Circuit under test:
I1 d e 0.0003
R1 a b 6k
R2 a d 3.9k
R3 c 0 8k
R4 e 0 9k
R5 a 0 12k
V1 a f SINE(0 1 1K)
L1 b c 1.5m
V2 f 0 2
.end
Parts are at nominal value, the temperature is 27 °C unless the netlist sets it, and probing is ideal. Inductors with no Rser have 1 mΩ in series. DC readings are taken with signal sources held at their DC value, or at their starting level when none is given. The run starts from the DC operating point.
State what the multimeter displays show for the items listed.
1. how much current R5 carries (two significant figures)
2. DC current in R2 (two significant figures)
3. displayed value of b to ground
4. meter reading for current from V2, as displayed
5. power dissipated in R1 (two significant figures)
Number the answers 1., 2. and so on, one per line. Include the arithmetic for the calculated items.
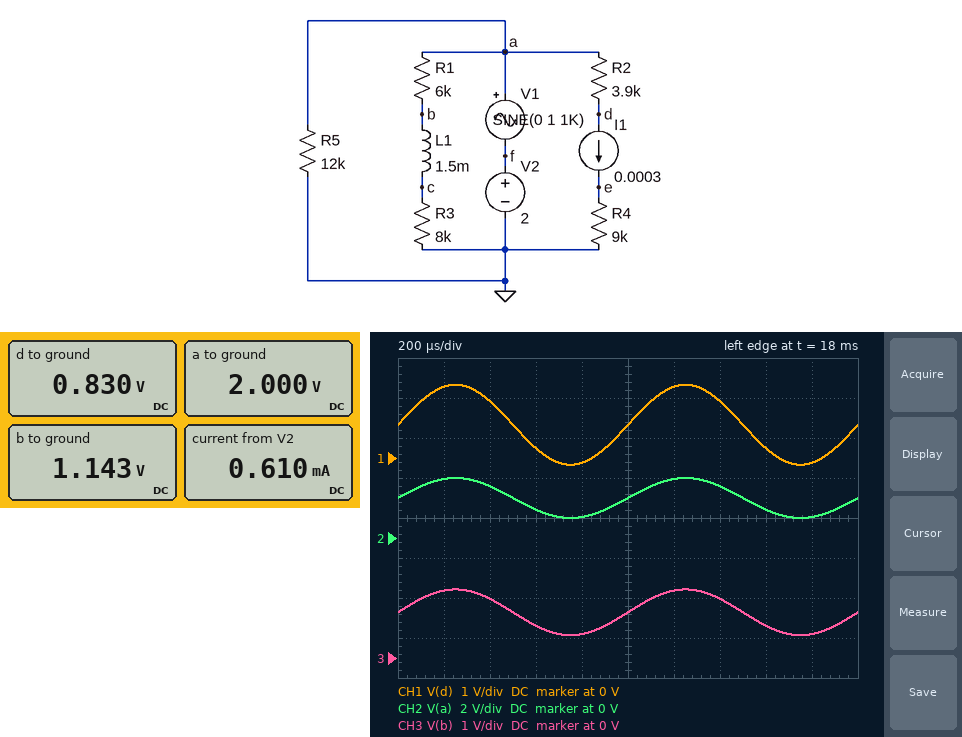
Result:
1. (2 V) / 12 kΩ = 170 µA
2. (2 V - 830 mV) / 3.9 kΩ = 300 µA
3. 1.143 V
4. 0.610 mA
5. (2 V - 1.143 V)^2 / 6 kΩ = 120 µW
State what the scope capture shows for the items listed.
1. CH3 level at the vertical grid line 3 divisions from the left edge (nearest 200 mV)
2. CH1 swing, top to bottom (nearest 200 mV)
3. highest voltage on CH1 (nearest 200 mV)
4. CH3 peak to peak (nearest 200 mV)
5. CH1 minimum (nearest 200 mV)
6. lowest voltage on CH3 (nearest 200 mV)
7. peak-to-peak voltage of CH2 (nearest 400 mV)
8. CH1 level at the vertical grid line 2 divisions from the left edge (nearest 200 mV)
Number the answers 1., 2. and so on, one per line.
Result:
1. 800 mV
2. 2.0 V
3. 1.8 V
4. 1.2 V
5. -200 mV
6. 600 mV
7. 2.0 V
8. 1.4 V
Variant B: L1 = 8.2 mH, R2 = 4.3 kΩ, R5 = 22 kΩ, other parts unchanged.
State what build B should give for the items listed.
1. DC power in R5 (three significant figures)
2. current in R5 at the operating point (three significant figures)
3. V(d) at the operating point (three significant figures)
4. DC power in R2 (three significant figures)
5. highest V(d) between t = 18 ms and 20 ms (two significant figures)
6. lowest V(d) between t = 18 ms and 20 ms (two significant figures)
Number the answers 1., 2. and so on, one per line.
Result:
1. 182 µW
2. 90.9 µA
3. 710 mV
4. 387 µW
5. 1.7 V
6. -290 mV
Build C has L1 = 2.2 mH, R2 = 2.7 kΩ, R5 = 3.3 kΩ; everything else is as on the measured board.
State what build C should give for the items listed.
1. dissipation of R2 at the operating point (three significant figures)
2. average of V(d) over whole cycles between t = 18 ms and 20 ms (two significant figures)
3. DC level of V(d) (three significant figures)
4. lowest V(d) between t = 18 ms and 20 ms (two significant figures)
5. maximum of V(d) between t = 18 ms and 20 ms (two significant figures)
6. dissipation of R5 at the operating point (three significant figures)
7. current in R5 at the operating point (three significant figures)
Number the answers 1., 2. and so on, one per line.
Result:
1. 243 µW
2. 1.2 V
3. 1.19 V
4. 190 mV
5. 2.2 V
6. 1.21 mW
7. 606 µA
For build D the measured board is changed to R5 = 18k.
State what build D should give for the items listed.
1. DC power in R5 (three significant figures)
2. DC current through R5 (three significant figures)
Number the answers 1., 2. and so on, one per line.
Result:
1. 222 µW
2. 111 µA
